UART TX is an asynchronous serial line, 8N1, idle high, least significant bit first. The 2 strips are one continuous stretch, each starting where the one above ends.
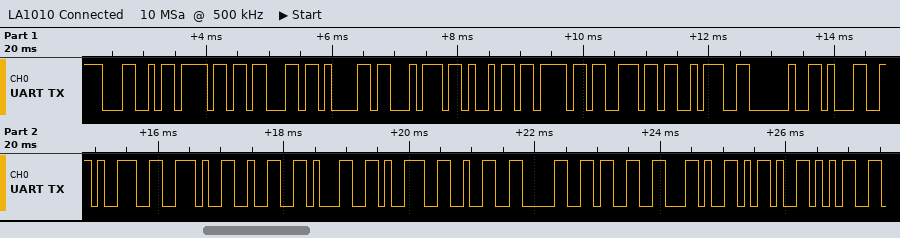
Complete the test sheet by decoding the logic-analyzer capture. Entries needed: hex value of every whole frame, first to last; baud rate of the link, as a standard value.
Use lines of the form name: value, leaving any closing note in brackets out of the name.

hex value of every whole frame, first to last: 0x4C 0x6F 0x63 0x61 0x74 0x69 0x6F 0x6E 0x3A 0x20 0x31 0x39 0x2E 0x32 0x31 0x39 0x32 0x30 0x33 0x2C 0x2D 0x35
baud rate of the link, as a standard value: 9600 baud
